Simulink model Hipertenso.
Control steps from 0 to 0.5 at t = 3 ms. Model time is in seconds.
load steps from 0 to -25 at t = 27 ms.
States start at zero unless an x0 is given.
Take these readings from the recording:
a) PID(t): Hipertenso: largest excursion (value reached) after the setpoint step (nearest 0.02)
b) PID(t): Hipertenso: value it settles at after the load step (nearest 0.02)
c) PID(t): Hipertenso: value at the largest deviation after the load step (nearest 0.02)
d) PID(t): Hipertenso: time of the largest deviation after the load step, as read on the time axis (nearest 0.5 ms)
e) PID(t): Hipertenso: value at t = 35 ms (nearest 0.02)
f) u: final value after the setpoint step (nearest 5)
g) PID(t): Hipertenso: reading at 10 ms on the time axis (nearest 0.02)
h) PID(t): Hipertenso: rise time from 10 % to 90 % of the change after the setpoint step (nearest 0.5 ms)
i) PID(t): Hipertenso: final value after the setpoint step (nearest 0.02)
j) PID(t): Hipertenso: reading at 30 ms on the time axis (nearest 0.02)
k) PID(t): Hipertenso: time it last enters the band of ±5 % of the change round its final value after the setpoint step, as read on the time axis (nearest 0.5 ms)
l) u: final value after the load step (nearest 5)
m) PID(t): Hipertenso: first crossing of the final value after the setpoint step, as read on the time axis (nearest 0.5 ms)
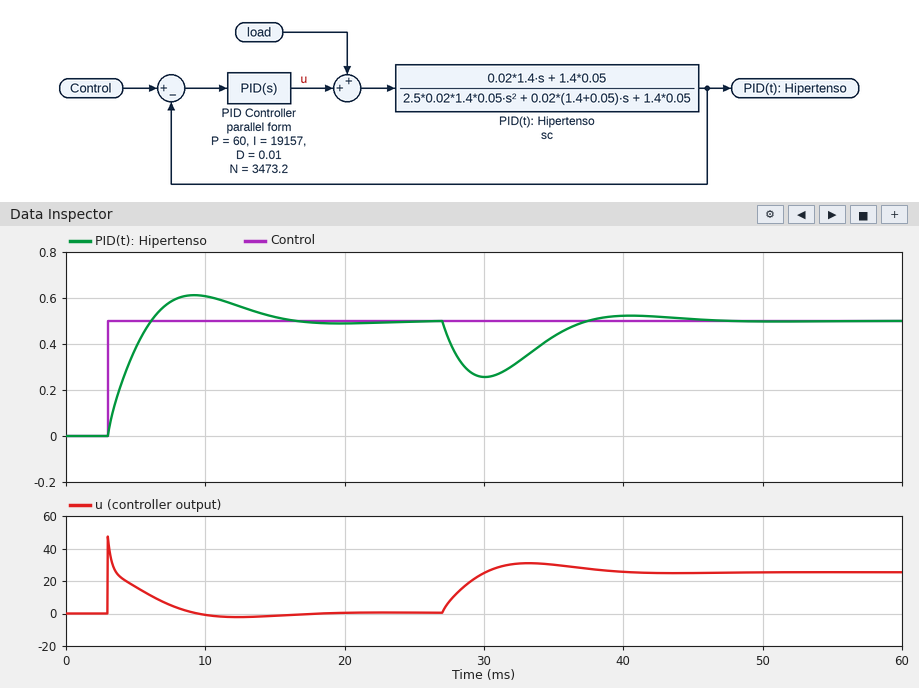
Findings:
0.62
0.50
0.26
30.0 ms
0.44
0
0.60
2.5 ms
0.50
0.26
14.5 ms
25
6.0 ms
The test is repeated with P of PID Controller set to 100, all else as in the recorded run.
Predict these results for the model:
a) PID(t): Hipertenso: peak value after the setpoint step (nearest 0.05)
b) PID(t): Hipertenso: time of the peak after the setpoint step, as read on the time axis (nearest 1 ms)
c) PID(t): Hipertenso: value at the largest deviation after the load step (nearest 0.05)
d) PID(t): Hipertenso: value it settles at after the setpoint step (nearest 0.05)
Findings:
0.55
8 ms
0.30
0.50
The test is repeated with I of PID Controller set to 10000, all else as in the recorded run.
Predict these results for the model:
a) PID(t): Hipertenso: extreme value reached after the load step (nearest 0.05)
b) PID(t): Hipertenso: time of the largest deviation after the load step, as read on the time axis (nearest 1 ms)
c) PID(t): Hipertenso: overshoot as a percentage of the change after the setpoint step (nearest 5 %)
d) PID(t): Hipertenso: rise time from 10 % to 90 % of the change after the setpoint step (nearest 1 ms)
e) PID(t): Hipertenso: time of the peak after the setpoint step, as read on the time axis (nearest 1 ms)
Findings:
0.20
31 ms
15 %
3 ms
11 ms
